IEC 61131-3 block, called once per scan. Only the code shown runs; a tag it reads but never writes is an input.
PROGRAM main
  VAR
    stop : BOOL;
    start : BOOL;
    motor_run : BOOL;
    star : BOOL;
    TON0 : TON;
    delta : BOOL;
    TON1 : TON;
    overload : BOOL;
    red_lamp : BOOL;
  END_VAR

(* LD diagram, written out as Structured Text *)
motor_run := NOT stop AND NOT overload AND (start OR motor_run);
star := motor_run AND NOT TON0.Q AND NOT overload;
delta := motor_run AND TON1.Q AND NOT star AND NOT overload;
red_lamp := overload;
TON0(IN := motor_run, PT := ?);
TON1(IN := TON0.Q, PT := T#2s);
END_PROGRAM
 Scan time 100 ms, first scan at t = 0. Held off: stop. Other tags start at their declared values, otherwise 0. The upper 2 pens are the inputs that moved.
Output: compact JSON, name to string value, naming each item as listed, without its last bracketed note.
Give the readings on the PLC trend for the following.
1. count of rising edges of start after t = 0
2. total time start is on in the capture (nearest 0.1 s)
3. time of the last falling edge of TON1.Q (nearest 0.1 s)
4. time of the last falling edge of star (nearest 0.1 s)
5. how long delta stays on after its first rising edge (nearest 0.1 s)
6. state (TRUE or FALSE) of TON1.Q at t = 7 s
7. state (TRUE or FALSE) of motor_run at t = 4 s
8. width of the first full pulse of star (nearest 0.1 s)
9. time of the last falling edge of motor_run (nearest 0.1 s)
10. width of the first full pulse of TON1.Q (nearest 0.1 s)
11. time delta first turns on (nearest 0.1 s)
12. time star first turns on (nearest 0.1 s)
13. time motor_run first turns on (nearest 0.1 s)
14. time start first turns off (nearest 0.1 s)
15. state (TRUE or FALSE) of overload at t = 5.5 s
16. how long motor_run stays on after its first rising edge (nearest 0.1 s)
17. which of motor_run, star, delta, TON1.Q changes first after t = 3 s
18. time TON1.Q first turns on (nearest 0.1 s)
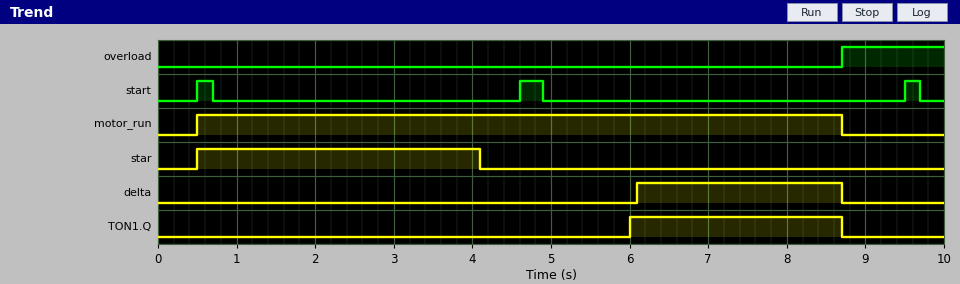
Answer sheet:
{"count of rising edges of start after t = 0": "3", "total time start is on in the capture": "0.7 s", "time of the last falling edge of TON1.Q": "8.7 s", "time of the last falling edge of star": "4.1 s", "how long delta stays on after its first rising edge": "2.6 s", "state (TRUE or FALSE) of TON1.Q at t = 7 s": "TRUE", "state (TRUE or FALSE) of motor_run at t = 4 s": "TRUE", "width of the first full pulse of star": "3.6 s", "time of the last falling edge of motor_run": "8.7 s", "width of the first full pulse of TON1.Q": "2.7 s", "time delta first turns on": "6.1 s", "time star first turns on": "0.5 s", "time motor_run first turns on": "0.5 s", "time start first turns off": "0.7 s", "state (TRUE or FALSE) of overload at t = 5.5 s": "FALSE", "how long motor_run stays on after its first rising edge": "8.2 s", "which of motor_run, star, delta, TON1.Q changes first after t = 3 s": "star", "time TON1.Q first turns on": "6.0 s"}
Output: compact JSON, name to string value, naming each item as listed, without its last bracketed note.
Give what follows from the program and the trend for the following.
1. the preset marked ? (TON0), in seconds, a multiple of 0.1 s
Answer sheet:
{"the preset marked ? (TON0), in seconds, a multiple of 0.1 s": "3.5 s"}
